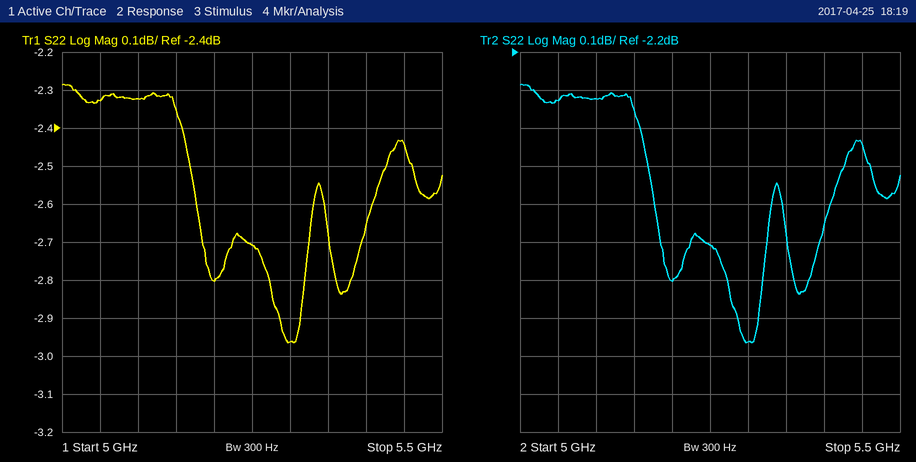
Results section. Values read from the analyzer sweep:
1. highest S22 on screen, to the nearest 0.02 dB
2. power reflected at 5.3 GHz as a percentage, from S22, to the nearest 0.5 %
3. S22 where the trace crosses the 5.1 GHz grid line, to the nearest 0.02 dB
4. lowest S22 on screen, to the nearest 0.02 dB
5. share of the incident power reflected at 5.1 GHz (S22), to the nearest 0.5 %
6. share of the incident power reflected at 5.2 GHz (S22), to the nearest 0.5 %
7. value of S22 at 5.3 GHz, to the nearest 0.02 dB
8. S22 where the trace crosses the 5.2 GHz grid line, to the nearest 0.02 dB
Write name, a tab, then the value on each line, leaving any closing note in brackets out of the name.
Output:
highest S22 on screen, to the nearest 0.02 dB	-2.28 dB
power reflected at 5.3 GHz as a percentage, from S22, to the nearest 0.5 %	50.5 %
S22 where the trace crosses the 5.1 GHz grid line, to the nearest 0.02 dB	-2.32 dB
lowest S22 on screen, to the nearest 0.02 dB	-2.96 dB
share of the incident power reflected at 5.1 GHz (S22), to the nearest 0.5 %	58.5 %
share of the incident power reflected at 5.2 GHz (S22), to the nearest 0.5 %	52.5 %
value of S22 at 5.3 GHz, to the nearest 0.02 dB	-2.96 dB
S22 where the trace crosses the 5.2 GHz grid line, to the nearest 0.02 dB	-2.80 dB
